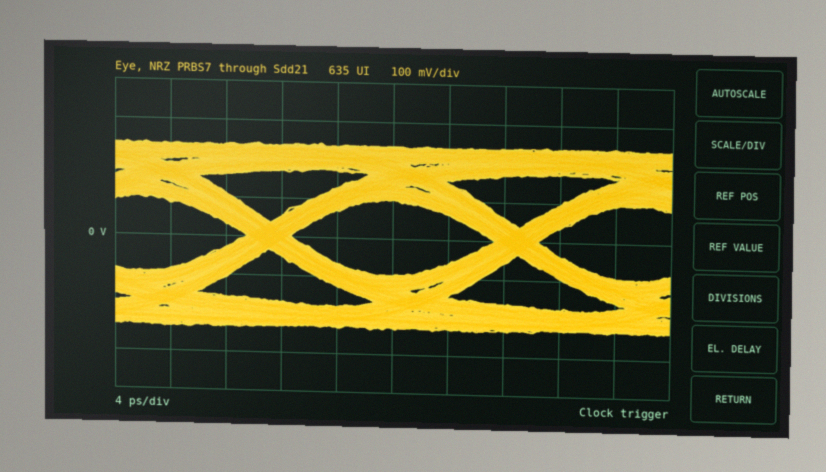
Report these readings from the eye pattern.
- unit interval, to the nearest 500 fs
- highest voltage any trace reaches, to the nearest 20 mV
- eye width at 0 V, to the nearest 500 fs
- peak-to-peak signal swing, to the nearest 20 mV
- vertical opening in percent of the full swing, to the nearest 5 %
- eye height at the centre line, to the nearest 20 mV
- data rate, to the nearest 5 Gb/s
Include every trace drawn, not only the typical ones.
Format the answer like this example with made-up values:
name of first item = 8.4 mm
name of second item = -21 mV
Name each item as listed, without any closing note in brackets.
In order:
unit interval, to the nearest 500 fs = 18.0 ps
highest voltage any trace reaches, to the nearest 20 mV = 240 mV
eye width at 0 V, to the nearest 500 fs = 14.5 ps
peak-to-peak signal swing, to the nearest 20 mV = 480 mV
vertical opening in percent of the full swing, to the nearest 5 % = 40 %
eye height at the centre line, to the nearest 20 mV = 200 mV
data rate, to the nearest 5 Gb/s = 55 Gb/s
